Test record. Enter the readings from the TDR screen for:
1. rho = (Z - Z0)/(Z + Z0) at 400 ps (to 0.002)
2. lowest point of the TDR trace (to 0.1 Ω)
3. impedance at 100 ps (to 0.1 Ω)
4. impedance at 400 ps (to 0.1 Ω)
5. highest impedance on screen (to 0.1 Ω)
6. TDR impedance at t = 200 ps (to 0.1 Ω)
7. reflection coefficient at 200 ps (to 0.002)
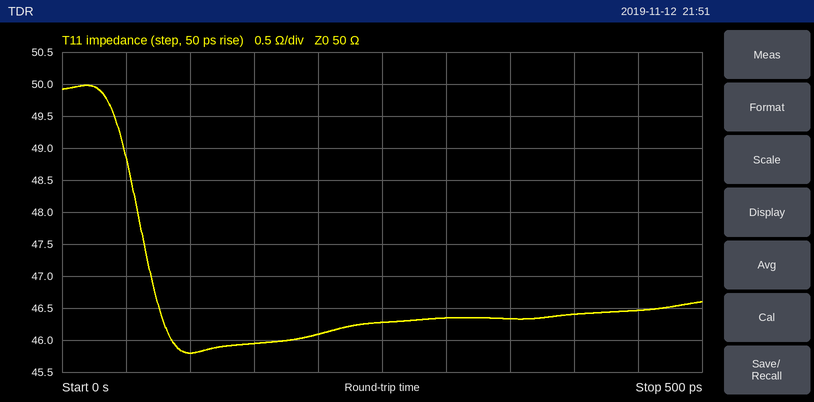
-0.038
45.8 Ω
45.8 Ω
46.4 Ω
50.0 Ω
46.1 Ω
-0.040
